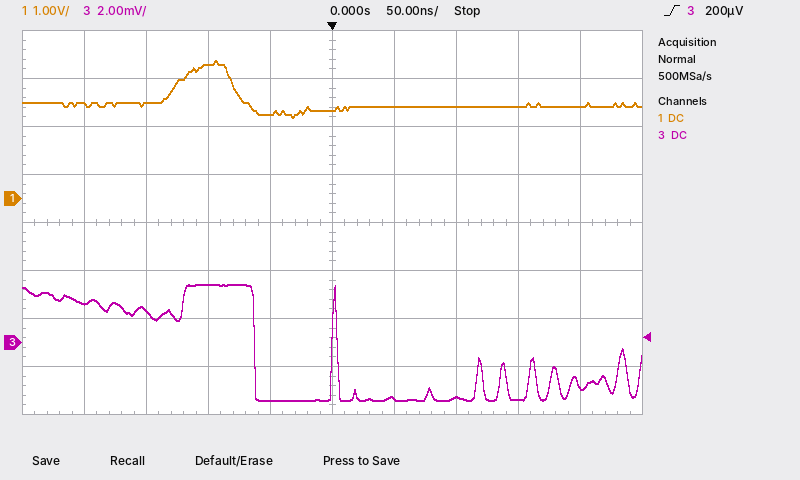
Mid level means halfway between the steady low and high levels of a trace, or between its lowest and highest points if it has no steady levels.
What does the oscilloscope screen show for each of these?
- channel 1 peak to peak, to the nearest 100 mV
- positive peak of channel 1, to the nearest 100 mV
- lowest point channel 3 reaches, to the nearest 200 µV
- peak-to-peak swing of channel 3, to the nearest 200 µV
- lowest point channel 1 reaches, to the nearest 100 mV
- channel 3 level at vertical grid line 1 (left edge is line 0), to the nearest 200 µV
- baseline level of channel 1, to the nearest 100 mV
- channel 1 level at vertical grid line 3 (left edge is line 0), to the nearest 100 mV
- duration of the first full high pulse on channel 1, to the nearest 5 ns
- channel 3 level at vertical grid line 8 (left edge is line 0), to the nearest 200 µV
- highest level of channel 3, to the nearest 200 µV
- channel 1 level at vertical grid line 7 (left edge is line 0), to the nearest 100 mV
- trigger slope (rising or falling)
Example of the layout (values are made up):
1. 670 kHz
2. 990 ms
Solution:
1. 1.2 V
2. 2.9 V
3. -2.4 mV
4. 4.8 mV
5. 1.7 V
6. 1.6 mV
7. 1.9 V
8. 2.8 V
9. 50 ns
10. -2.4 mV
11. 2.4 mV
12. 1.9 V
13. rising
